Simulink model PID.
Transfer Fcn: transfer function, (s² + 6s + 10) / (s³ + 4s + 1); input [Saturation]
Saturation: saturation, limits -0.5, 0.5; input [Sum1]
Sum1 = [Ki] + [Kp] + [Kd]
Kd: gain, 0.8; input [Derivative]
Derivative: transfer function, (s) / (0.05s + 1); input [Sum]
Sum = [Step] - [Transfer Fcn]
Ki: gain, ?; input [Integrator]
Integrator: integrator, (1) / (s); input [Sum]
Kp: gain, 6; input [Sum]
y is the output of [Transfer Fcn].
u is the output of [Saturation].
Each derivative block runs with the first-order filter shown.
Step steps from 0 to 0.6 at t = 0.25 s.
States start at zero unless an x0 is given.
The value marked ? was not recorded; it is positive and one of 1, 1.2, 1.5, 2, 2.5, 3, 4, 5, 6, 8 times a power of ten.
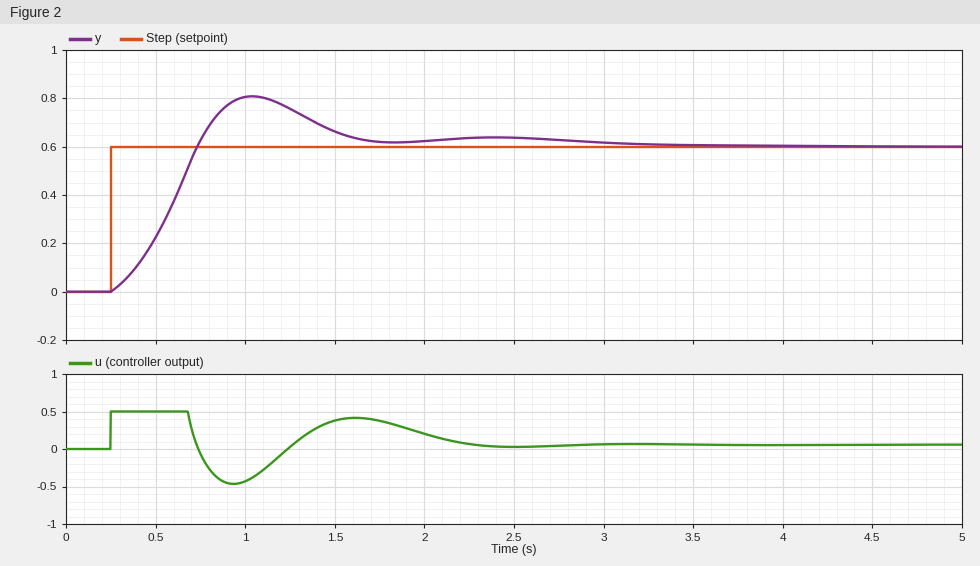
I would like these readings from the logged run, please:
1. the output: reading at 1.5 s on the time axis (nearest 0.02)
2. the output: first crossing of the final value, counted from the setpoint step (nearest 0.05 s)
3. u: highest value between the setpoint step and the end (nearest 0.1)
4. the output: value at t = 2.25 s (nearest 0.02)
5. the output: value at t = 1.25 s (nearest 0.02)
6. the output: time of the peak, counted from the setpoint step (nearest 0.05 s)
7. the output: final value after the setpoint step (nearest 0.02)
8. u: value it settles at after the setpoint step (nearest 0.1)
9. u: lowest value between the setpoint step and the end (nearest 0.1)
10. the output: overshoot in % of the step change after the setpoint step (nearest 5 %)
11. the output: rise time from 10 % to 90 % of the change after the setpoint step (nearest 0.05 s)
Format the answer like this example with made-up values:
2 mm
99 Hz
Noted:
0.66
0.50 s
0.5
0.64
0.76
0.80 s
0.60
0.1
-0.5
35 %
0.35 s
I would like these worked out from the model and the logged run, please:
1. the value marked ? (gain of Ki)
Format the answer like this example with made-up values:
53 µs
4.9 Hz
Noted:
8
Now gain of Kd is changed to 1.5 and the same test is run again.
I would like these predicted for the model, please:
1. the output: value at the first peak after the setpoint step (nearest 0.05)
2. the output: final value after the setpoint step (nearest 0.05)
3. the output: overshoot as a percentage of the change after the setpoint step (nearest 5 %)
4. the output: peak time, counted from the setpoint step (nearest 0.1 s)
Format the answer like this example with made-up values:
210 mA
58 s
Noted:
0.75
0.60
25 %
0.9 s
